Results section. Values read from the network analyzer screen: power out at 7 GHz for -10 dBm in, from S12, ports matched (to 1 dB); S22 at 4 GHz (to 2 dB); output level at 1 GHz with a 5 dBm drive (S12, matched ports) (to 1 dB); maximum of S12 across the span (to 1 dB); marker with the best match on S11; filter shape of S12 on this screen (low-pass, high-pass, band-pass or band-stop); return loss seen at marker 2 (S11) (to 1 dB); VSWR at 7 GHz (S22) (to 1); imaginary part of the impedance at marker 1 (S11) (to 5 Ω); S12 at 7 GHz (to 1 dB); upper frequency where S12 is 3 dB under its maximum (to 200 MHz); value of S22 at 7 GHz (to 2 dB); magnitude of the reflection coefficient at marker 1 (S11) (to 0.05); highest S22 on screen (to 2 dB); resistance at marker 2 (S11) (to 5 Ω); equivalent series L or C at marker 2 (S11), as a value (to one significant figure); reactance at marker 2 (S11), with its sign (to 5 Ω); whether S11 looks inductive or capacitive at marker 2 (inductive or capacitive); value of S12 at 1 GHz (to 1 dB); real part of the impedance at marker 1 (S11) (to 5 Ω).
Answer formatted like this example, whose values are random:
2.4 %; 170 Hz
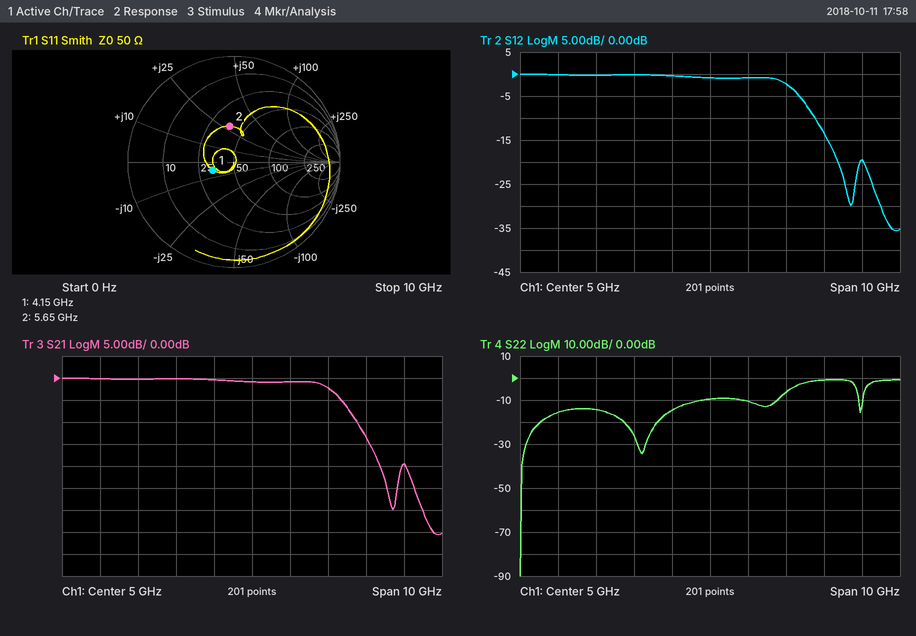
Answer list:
-12 dBm; -14 dB; 5 dBm; 0 dB; marker 1; low-pass; 9 dB; 3; -5 Ω; -2 dB; 7.2 GHz; -6 dB; 0.20; 0 dB; 35 Ω; 800 pH; +30 Ω; inductive; 0 dB; 35 Ω
